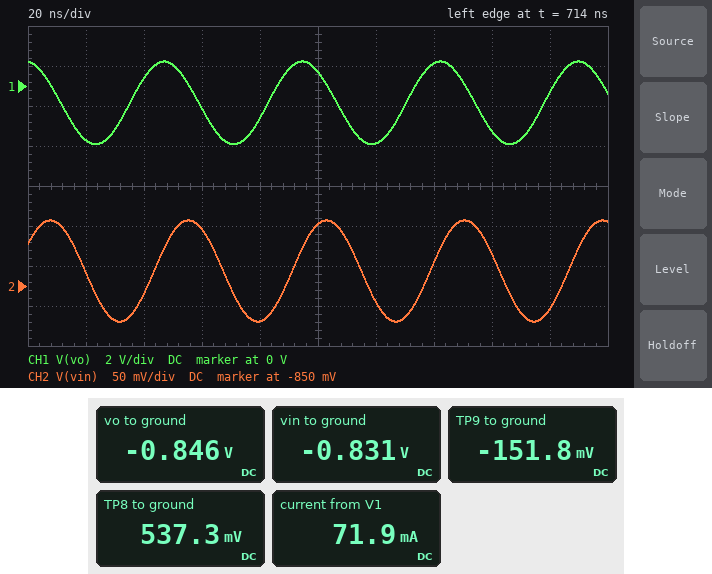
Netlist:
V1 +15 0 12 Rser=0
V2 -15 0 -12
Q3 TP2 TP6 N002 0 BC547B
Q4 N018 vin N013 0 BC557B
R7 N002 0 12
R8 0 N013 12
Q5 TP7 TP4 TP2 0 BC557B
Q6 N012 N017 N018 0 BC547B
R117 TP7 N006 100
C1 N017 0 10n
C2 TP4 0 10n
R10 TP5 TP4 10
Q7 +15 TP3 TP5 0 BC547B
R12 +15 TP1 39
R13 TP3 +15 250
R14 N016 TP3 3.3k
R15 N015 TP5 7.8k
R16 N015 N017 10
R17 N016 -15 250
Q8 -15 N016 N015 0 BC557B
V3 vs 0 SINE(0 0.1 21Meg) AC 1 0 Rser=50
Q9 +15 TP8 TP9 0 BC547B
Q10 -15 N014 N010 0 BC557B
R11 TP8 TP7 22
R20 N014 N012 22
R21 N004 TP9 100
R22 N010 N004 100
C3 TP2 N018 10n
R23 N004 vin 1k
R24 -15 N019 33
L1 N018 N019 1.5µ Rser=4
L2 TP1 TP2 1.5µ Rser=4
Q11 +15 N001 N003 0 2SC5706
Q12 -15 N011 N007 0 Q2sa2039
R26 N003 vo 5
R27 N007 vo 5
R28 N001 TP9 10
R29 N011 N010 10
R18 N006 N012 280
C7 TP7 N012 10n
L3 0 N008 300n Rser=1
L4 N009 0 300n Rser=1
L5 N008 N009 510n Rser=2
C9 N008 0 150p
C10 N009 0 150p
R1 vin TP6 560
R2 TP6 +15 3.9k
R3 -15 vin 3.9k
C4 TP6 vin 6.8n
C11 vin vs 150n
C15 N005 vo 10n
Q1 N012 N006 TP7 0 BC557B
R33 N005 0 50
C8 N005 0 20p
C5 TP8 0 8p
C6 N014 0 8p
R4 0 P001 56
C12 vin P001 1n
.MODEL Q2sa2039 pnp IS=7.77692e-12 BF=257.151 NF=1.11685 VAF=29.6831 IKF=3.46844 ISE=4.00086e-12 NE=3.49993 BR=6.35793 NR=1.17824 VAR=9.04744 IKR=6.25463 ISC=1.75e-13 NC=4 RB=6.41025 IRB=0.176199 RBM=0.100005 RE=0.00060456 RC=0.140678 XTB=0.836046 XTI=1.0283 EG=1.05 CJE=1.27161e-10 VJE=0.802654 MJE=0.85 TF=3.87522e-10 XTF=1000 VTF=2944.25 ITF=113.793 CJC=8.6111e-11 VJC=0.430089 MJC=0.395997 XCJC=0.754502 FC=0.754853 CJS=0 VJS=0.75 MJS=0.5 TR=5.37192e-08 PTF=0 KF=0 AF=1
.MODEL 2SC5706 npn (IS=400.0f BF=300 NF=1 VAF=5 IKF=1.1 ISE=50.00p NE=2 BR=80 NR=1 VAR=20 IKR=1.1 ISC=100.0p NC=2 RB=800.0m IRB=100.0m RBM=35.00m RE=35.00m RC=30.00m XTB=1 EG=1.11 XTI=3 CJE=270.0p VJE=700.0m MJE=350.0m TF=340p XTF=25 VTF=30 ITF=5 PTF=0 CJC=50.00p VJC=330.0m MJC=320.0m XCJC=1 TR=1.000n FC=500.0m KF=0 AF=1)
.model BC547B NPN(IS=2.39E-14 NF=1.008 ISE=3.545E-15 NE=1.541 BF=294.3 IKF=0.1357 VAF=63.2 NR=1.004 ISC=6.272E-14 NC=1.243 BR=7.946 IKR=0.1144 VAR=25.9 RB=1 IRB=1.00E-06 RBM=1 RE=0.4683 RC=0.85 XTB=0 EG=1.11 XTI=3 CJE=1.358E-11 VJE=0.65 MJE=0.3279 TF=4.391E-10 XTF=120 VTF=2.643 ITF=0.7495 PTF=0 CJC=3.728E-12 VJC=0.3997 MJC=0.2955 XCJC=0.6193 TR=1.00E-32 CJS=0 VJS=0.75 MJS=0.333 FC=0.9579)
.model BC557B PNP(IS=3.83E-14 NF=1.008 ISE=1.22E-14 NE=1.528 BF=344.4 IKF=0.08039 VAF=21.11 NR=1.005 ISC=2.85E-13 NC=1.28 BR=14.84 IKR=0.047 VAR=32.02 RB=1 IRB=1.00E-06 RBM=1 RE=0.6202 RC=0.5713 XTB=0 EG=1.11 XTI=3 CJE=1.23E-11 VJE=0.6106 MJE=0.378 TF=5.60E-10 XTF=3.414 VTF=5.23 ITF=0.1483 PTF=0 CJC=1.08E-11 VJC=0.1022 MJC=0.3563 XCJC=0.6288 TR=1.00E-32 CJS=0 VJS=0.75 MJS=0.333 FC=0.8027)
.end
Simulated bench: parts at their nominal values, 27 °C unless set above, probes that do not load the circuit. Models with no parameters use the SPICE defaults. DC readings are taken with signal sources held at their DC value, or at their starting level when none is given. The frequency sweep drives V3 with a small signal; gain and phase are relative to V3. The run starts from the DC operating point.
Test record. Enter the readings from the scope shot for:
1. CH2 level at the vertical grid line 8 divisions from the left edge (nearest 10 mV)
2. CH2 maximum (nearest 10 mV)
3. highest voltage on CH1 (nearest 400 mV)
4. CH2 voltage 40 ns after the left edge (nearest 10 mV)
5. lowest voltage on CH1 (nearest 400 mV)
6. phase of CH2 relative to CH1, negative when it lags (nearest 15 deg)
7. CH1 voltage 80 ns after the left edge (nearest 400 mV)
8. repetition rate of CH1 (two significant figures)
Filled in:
-810 mV
-770 mV
1.2 V
-860 mV
-2.8 V
-60 deg
-1.6 V
21 MHz
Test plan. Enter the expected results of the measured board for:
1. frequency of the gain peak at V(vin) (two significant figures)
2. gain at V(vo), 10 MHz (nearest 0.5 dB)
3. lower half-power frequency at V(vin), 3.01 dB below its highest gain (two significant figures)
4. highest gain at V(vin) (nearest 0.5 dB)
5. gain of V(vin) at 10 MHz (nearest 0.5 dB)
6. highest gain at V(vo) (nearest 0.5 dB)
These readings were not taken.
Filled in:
28 MHz
26.5 dB
16 MHz
-3.5 dB
-11.0 dB
27.0 dB
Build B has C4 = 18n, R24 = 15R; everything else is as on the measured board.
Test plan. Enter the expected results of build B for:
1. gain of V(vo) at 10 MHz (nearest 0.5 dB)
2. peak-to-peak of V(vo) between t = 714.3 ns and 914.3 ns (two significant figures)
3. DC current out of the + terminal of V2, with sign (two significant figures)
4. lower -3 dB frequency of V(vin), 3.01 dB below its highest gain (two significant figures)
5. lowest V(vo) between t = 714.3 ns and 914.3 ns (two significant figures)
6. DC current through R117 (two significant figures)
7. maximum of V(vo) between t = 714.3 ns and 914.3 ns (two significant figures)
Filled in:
25.5 dB
2.4 V
-120 mA
10 MHz
-2.8 V
7.3 mA
-400 mV
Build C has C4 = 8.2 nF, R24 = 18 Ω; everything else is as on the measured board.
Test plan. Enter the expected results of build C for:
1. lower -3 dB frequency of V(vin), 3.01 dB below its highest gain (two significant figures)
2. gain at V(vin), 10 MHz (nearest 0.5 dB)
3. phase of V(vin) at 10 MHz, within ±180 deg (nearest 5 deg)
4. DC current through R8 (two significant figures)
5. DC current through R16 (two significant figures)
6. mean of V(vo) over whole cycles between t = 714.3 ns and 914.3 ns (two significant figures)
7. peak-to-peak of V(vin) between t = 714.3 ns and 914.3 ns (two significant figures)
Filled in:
10 MHz
-7.5 dB
50 deg
32 mA
140 µA
-1.4 V
120 mV
